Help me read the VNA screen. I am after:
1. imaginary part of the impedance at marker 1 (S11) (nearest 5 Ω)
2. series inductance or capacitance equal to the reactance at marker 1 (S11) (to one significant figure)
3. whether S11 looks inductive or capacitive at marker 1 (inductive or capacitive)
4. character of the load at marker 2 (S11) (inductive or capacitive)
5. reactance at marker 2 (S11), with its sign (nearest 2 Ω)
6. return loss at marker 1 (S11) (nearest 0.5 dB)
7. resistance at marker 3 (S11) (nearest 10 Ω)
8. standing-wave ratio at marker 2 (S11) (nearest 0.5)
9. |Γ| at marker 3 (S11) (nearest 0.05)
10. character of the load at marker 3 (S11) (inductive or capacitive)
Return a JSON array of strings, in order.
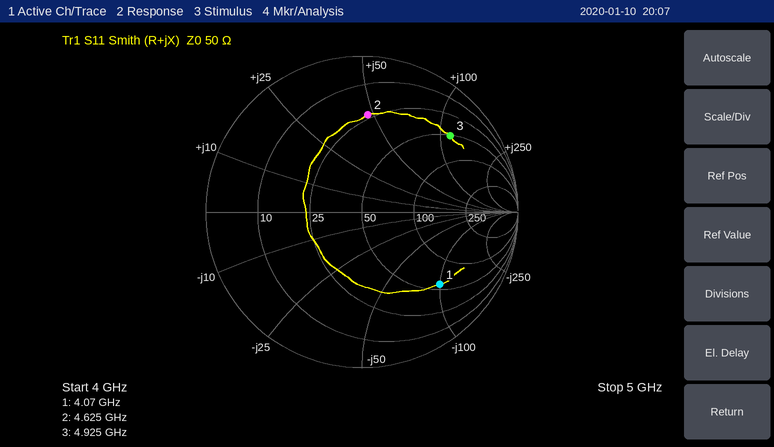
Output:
["-100 Ω", "400 fF", "capacitive", "inductive", "+48 Ω", "3.5 dB", "50 Ω", "4.5", "0.75", "inductive"]
